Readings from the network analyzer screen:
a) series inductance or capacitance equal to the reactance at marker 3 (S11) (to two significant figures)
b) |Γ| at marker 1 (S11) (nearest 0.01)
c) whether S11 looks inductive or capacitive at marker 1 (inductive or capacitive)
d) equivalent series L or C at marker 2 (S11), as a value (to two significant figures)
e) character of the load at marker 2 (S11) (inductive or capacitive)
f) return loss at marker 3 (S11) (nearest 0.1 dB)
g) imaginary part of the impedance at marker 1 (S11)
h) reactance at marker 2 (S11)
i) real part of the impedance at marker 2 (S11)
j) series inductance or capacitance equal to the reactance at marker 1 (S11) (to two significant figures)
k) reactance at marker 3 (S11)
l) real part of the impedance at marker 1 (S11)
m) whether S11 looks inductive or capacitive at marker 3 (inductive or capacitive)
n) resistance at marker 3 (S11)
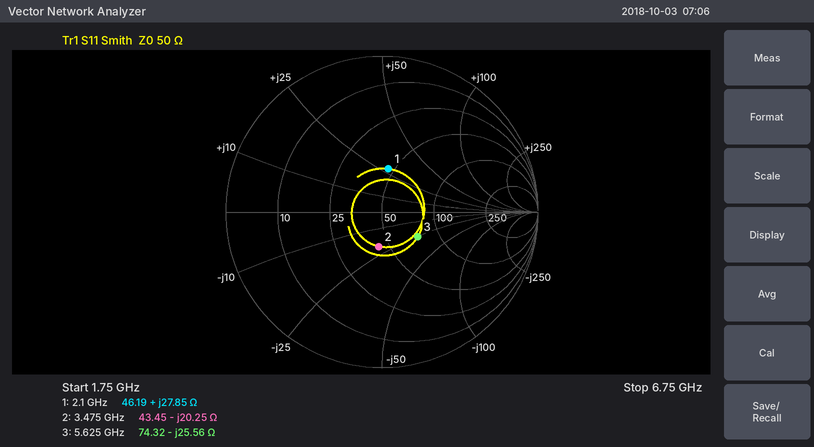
1.1 pF
0.28
inductive
2.3 pF
capacitive
11.1 dB
+27.85 Ω
-20.25 Ω
43.45 Ω
2.1 nH
-25.56 Ω
46.19 Ω
capacitive
74.32 Ω
